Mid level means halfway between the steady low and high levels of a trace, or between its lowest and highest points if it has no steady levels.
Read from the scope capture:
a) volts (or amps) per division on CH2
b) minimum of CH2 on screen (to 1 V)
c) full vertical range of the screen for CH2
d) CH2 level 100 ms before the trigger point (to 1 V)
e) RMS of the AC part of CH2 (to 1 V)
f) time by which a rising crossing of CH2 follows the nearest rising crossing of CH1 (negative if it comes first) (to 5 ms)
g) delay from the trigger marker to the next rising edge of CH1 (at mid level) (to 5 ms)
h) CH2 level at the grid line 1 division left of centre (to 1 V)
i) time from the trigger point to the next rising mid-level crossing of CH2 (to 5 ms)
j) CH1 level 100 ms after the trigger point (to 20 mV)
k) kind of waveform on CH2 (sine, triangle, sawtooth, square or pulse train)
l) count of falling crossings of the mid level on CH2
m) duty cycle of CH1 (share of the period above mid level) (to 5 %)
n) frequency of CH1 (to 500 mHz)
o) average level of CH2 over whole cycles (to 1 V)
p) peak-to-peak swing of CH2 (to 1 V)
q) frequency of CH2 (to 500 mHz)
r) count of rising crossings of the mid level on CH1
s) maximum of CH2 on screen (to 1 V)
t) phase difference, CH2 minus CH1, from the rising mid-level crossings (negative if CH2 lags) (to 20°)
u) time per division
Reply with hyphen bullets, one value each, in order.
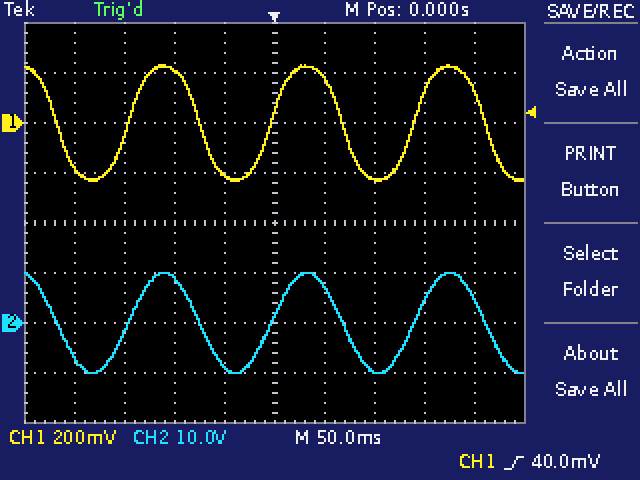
- 10 V
- -10 V
- 80 V
- 9 V
- 7 V
- 0 ms
- 140 ms
- -9 V
- 140 ms
- -220 mV
- sine
- 4
- 50 %
- 7.0 Hz
- 0 V
- 20 V
- 7.0 Hz
- 3
- 10 V
- 0°
- 50 ms
